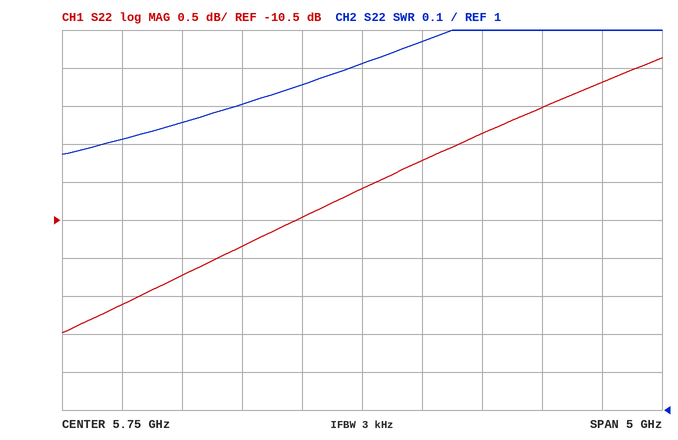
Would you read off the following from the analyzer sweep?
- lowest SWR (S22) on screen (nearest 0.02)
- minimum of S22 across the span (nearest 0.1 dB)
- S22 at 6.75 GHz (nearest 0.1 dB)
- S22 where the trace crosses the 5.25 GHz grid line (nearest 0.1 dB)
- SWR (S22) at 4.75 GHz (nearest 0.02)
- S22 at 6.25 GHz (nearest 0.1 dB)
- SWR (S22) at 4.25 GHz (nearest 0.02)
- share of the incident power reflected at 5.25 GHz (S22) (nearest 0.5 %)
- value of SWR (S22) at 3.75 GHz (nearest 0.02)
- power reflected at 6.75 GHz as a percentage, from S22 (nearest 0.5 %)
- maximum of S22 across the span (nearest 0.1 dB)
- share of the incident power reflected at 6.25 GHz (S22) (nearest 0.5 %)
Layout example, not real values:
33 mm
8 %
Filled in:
1.68
-12.0 dB
-9.4 dB
-10.5 dB
1.80
-9.7 dB
1.76
9.0 %
1.72
11.5 %
-8.4 dB
10.5 %
